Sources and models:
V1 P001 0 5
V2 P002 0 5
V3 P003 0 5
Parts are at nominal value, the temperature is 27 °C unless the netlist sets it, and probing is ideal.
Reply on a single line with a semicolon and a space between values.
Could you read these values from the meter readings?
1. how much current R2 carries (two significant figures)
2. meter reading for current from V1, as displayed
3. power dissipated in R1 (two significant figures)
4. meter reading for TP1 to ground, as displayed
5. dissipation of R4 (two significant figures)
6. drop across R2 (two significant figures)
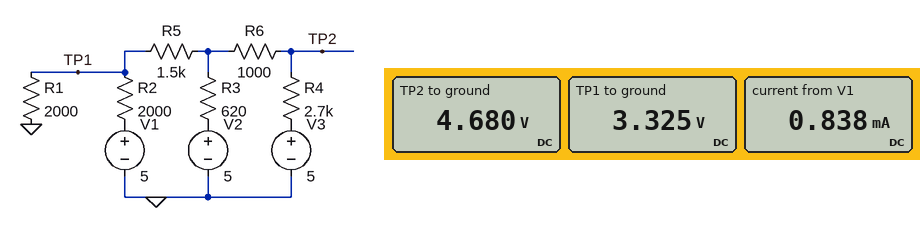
840 µA; 0.838 mA; 5.5 mW; 3.325 V; 38 µW; 1.7 V
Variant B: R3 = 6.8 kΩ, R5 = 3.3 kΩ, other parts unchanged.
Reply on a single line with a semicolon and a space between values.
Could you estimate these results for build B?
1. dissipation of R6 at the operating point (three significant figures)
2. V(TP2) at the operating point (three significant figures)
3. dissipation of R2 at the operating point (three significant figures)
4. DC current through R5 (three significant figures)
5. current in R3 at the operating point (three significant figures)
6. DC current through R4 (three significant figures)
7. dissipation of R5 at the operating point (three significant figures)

58.5 µW; 4.35 V; 2.26 mW; 373 µA; 132 µA; 242 µA; 460 µW
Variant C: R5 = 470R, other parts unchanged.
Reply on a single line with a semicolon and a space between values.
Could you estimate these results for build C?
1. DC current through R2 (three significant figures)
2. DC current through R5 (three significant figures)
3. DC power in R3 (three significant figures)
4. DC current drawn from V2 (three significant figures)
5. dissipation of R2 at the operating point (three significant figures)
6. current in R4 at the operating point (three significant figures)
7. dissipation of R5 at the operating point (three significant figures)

625 µA; 1.25 mA; 710 µW; 1.07 mA; 782 µW; 179 µA; 734 µW
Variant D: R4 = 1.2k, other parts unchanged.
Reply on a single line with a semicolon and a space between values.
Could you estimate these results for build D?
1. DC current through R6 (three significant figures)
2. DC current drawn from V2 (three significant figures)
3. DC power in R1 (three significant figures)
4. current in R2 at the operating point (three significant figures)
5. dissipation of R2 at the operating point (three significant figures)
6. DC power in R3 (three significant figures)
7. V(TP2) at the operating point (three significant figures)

184 µA; 654 µA; 5.57 mW; 831 µA; 1.38 mW; 265 µW; 4.78 V
